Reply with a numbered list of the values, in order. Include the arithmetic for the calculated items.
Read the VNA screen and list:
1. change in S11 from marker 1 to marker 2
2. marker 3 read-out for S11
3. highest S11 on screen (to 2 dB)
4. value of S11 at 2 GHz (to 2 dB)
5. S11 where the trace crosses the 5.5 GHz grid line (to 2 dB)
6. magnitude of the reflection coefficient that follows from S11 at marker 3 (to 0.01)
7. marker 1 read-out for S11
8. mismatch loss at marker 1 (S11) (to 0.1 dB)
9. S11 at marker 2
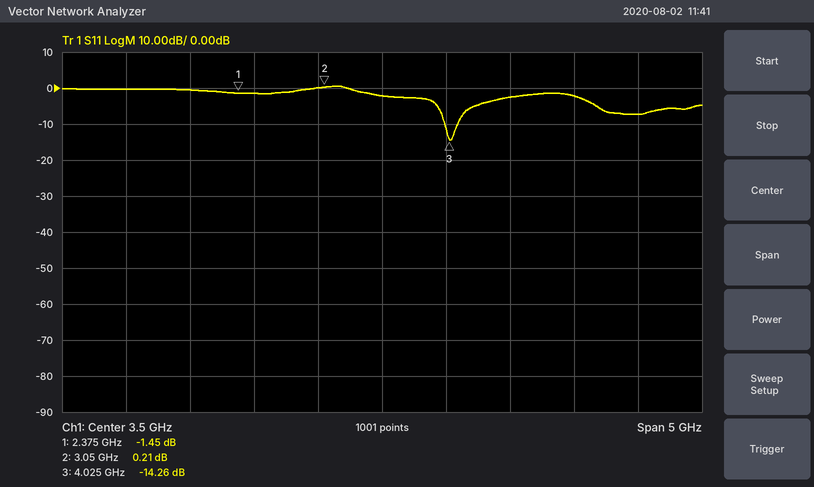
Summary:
1. 0.21 − (-1.45) = 1.66 dB
2. -14.26 dB
3. 0 dB
4. 0 dB
5. -8 dB
6. 10^(-14.26/20) ≈ 0.19
7. -1.45 dB
8. −10 log10(1 − 10^(-1.45/10)) ≈ 5.5 dB
9. 0.21 dB
